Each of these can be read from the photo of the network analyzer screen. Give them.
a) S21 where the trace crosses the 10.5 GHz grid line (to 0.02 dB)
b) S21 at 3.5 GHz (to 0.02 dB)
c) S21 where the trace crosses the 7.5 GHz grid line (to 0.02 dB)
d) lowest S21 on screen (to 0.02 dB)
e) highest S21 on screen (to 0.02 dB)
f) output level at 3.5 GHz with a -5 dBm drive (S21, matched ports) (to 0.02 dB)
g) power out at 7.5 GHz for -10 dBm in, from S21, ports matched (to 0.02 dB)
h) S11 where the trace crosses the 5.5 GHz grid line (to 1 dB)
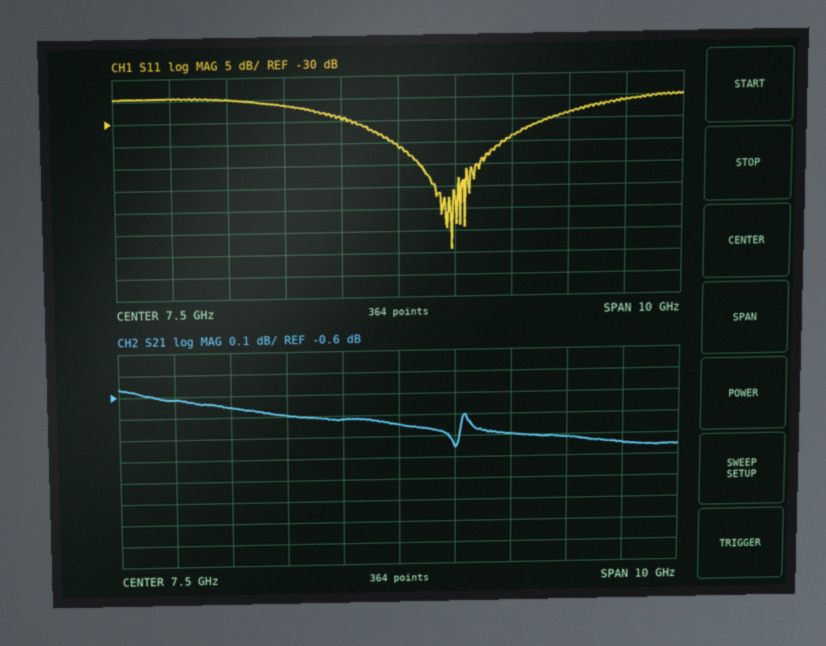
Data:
-0.82 dB
-0.62 dB
-0.74 dB
-0.86 dB
-0.56 dB
-5.62 dBm
-10.74 dBm
-26 dB
